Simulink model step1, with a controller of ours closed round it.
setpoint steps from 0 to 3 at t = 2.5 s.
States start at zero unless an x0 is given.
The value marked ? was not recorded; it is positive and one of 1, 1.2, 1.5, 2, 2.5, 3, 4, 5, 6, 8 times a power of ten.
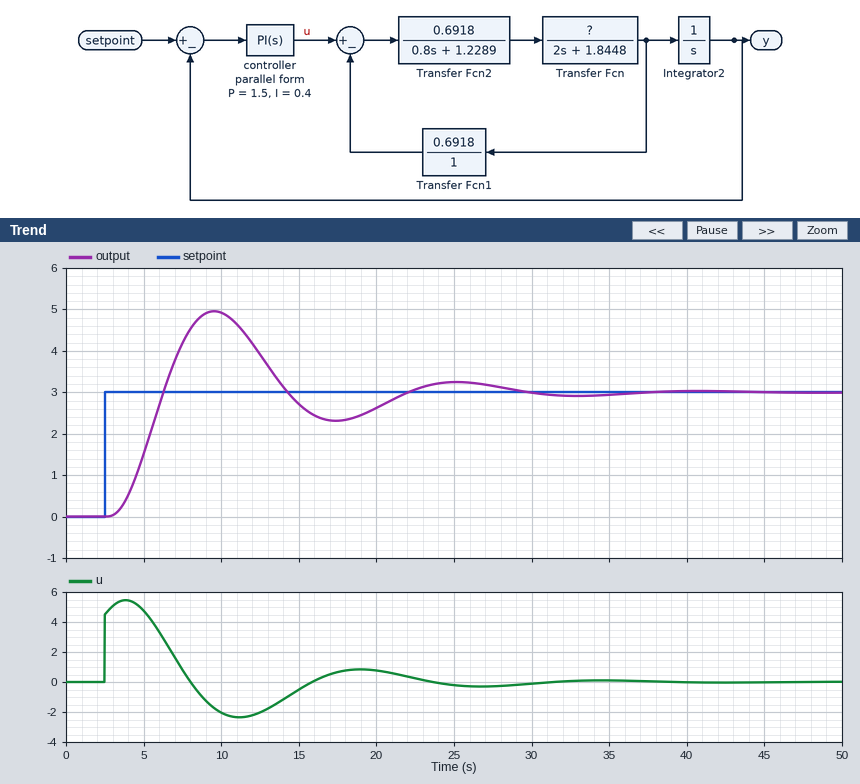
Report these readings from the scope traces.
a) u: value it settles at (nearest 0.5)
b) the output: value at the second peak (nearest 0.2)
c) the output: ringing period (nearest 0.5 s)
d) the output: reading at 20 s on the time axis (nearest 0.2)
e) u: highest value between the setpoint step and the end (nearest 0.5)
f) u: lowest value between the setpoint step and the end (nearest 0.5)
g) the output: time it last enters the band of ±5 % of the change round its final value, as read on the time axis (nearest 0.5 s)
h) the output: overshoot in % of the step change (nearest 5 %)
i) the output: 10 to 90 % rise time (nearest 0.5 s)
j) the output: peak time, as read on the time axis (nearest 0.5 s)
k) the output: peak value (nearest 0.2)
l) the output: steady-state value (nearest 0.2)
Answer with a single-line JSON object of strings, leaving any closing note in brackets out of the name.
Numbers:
{"u: value it settles at": "0.0", "the output: value at the second peak": "3.2", "the output: ringing period": "15.5 s", "the output: reading at 20 s on the time axis": "2.6", "u: highest value between the setpoint step and the end": "5.5", "u: lowest value between the setpoint step and the end": "-2.5", "the output: time it last enters the band of ±5 % of the change round its final value, as read on the time axis": "27.5 s", "the output: overshoot in % of the step change": "65 %", "the output: 10 to 90 % rise time": "2.5 s", "the output: peak time, as read on the time axis": "9.5 s", "the output: peak value": "5.0", "the output: steady-state value": "3.0"}
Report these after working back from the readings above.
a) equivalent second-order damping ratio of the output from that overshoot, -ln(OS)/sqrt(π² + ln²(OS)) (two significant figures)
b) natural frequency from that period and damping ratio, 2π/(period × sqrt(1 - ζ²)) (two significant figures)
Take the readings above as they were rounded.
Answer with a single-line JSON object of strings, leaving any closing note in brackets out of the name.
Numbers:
{"equivalent second-order damping ratio of the output from that overshoot, -ln(OS)/sqrt(π² + ln²(OS))": "0.14", "natural frequency from that period and damping ratio, 2π/(period × sqrt(1 - ζ²))": "0.41 rad/s"}
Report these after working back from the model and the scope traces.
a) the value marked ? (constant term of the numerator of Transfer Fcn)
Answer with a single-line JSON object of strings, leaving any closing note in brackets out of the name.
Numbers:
{"the value marked ?": "1"}
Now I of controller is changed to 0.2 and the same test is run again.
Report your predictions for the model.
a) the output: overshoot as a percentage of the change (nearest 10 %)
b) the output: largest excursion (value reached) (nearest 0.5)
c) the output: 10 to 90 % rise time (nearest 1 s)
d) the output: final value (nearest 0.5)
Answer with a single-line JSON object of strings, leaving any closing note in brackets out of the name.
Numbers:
{"the output: overshoot as a percentage of the change": "40 %", "the output: largest excursion (value reached)": "4.0", "the output: 10 to 90 % rise time": "3 s", "the output: final value": "3.0"}
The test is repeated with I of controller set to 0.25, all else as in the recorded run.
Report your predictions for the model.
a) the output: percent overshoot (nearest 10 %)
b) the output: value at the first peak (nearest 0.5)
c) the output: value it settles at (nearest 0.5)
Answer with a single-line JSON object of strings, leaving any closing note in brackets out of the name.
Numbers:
{"the output: percent overshoot": "50 %", "the output: value at the first peak": "4.5", "the output: value it settles at": "3.0"}
